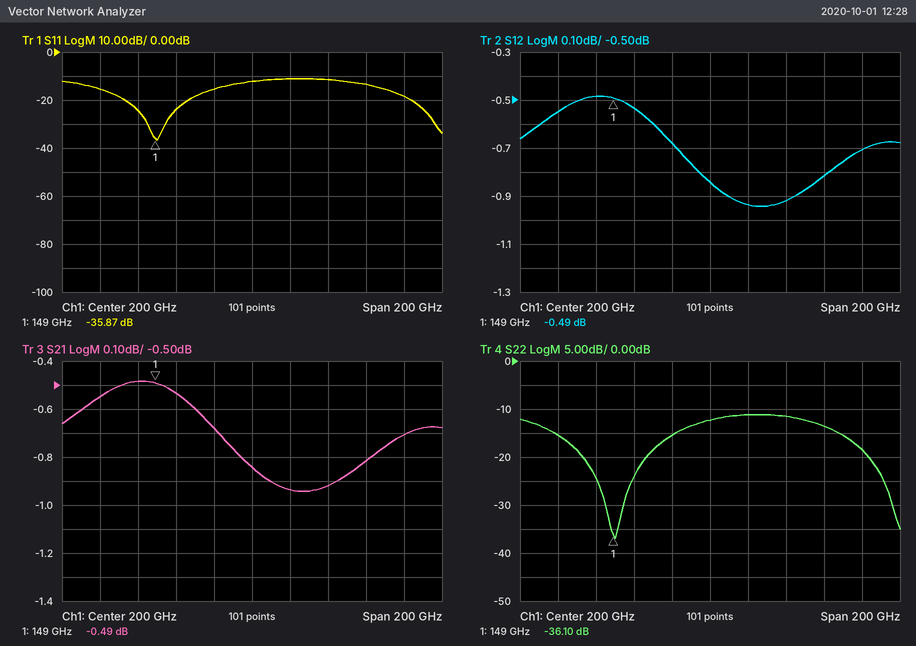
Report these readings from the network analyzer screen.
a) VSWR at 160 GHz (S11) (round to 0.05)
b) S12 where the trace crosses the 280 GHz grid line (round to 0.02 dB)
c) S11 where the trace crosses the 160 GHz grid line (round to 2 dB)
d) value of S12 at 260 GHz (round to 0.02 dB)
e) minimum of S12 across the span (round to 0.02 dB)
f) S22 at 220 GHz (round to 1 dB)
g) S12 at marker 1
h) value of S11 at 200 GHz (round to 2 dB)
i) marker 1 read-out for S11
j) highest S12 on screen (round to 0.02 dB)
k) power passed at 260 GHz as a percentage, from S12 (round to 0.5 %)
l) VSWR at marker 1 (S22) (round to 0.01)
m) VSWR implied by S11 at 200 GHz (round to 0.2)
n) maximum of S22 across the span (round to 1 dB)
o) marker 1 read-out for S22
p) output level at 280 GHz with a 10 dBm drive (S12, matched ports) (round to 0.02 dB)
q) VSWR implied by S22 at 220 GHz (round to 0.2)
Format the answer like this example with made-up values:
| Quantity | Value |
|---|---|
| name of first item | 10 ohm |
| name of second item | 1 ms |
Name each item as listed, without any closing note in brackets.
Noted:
| Quantity | Value |
|---|---|
| VSWR at 160 GHz (S11) | 1.15 |
| S12 where the trace crosses the 280 GHz grid line | -0.70 dB |
| S11 where the trace crosses the 160 GHz grid line | -24 dB |
| value of S12 at 260 GHz | -0.82 dB |
| minimum of S12 across the span | -0.94 dB |
| S22 at 220 GHz | -11 dB |
| S12 at marker 1 | -0.49 dB |
| value of S11 at 200 GHz | -12 dB |
| marker 1 read-out for S11 | -35.87 dB |
| highest S12 on screen | -0.48 dB |
| power passed at 260 GHz as a percentage, from S12 | 83.0 % |
| VSWR at marker 1 (S22) | 1.03 |
| VSWR implied by S11 at 200 GHz | 1.6 |
| maximum of S22 across the span | -11 dB |
| marker 1 read-out for S22 | -36.10 dB |
| output level at 280 GHz with a 10 dBm drive (S12, matched ports) | 9.30 dBm |
| VSWR implied by S22 at 220 GHz | 1.8 |
